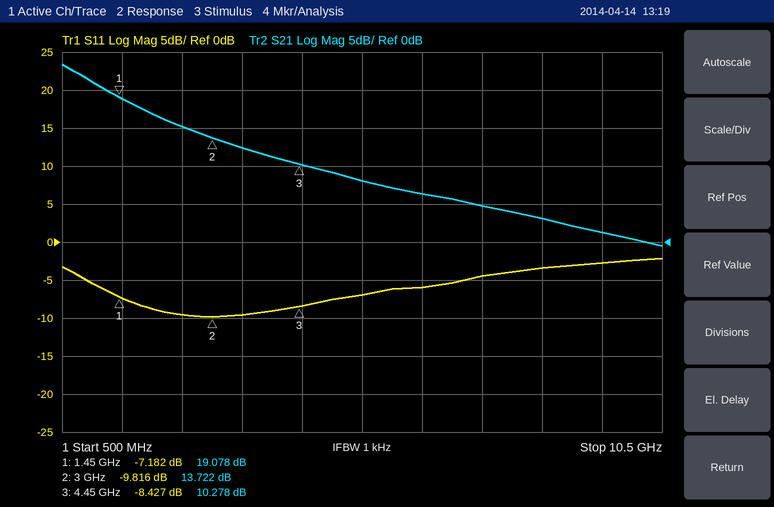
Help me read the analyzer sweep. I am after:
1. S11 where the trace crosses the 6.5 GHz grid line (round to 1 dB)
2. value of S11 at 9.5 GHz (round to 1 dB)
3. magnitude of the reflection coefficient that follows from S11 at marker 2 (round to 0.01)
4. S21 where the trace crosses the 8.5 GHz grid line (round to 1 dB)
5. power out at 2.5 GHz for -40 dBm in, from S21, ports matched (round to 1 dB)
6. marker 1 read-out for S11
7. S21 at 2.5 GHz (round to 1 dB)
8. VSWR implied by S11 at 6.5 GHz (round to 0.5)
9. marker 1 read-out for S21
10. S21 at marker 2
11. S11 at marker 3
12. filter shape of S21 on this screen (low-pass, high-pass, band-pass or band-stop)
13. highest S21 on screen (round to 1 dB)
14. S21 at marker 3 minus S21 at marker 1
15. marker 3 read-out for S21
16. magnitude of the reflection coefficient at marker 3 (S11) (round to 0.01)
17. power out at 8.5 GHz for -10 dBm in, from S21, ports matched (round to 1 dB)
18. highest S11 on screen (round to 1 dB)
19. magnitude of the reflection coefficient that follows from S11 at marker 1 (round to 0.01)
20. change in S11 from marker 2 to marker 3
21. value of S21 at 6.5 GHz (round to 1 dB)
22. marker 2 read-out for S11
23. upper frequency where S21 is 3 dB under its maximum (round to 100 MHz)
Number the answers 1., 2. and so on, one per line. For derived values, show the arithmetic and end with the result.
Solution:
1. -6 dB
2. -3 dB
3. 10^(-9.816/20) ≈ 0.32
4. 3 dB
5. -40 dBm + (15 dB) = -25 dBm
6. -7.182 dB
7. 15 dB
8. |Γ| = 10^(-6/20) = 0.5012; VSWR = (1 + 0.5012)/(1 − 0.5012) ≈ 3.0
9. 19.078 dB
10. 13.722 dB
11. -8.427 dB
12. low-pass
13. 23 dB
14. 10.278 − (19.078) = -8.800 dB
15. 10.278 dB
16. 10^(-8.427/20) ≈ 0.38
17. -10 dBm + (3 dB) = -7 dBm
18. -2 dB
19. 10^(-7.182/20) ≈ 0.44
20. -8.427 − (-9.816) = 1.389 dB
21. 6 dB
22. -9.816 dB
23. 1.2 GHz
